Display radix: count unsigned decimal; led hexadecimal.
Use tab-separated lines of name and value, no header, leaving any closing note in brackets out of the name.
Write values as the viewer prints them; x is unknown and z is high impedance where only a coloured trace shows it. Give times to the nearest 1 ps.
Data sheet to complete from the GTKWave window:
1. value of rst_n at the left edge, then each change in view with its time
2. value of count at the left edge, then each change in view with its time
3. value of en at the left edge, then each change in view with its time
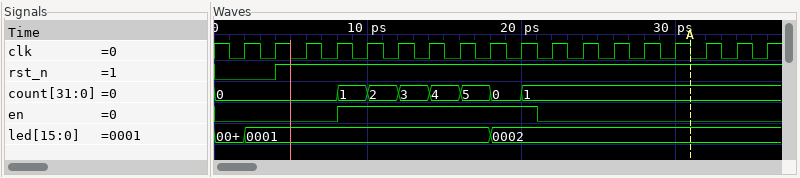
value of rst_n at the left edge, then each change in view with its time	0, 1 at 4 ps
value of count at the left edge, then each change in view with its time	0, 1 at 8 ps, 2 at 10 ps, 3 at 12 ps, 4 at 14 ps, 5 at 16 ps, 0 at 18 ps, 1 at 20 ps
value of en at the left edge, then each change in view with its time	0, 1 at 8 ps, 0 at 21 ps
